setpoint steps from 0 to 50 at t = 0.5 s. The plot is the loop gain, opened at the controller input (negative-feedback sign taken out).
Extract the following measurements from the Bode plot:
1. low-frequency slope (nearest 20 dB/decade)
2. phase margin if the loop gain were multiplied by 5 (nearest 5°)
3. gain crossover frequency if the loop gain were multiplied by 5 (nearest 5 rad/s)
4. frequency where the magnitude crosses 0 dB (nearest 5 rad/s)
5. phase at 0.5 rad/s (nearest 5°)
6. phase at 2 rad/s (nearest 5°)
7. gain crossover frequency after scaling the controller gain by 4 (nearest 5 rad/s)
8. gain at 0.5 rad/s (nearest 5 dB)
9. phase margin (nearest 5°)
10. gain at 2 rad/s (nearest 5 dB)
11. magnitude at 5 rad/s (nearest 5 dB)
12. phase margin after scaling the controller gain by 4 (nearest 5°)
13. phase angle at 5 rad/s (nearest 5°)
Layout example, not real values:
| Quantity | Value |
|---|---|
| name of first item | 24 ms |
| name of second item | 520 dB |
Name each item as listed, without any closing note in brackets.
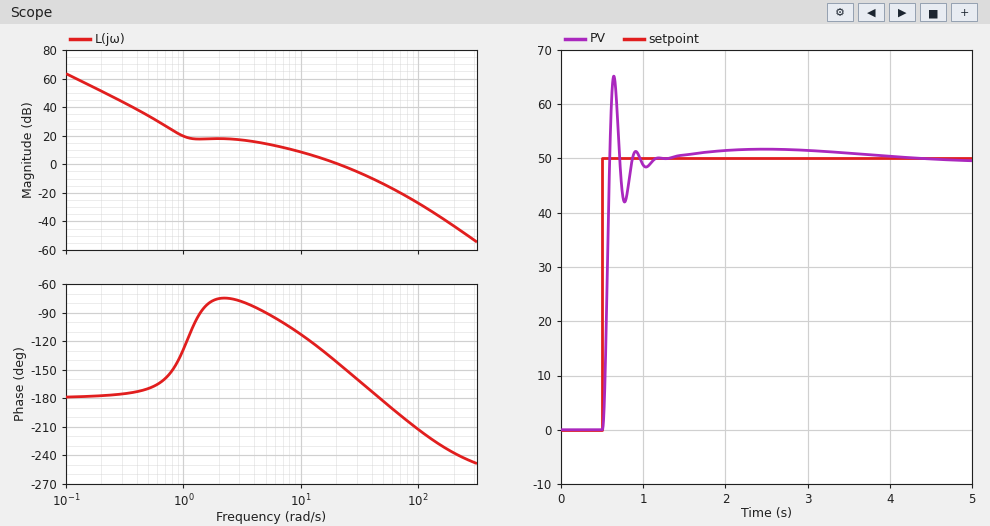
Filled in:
| Quantity | Value |
|---|---|
| low-frequency slope | -40 dB/decade |
| phase margin if the loop gain were multiplied by 5 | -5° |
| gain crossover frequency if the loop gain were multiplied by 5 | 50 rad/s |
| frequency where the magnitude crosses 0 dB | 20 rad/s |
| phase at 0.5 rad/s | -170° |
| phase at 2 rad/s | -75° |
| gain crossover frequency after scaling the controller gain by 4 | 45 rad/s |
| gain at 0.5 rad/s | 35 dB |
| phase margin | 35° |
| gain at 2 rad/s | 20 dB |
| magnitude at 5 rad/s | 15 dB |
| phase margin after scaling the controller gain by 4 | 0° |
| phase angle at 5 rad/s | -90° |
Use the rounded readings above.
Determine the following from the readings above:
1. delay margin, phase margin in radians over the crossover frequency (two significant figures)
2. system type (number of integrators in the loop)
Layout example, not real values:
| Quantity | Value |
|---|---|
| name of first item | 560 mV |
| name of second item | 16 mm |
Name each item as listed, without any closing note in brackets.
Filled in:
| Quantity | Value |
|---|---|
| delay margin, phase margin in radians over the crossover frequency | 0.031 s |
| system type | 2 |
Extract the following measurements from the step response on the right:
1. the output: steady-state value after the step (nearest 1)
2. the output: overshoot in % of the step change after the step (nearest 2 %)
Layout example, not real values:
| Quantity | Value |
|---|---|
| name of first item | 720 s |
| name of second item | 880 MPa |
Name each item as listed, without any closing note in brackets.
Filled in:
| Quantity | Value |
|---|---|
| the output: steady-state value after the step | 50 |
| the output: overshoot in % of the step change after the step | 30 % |
